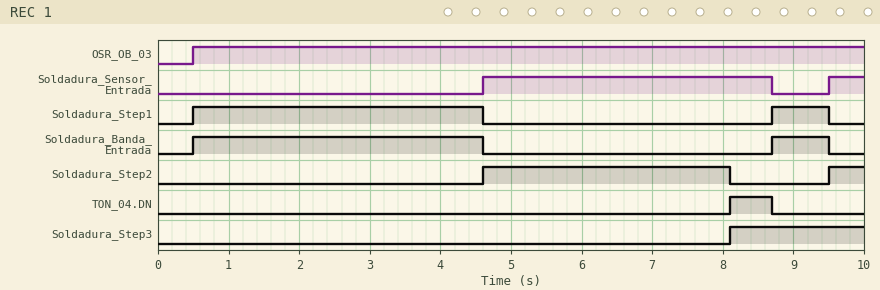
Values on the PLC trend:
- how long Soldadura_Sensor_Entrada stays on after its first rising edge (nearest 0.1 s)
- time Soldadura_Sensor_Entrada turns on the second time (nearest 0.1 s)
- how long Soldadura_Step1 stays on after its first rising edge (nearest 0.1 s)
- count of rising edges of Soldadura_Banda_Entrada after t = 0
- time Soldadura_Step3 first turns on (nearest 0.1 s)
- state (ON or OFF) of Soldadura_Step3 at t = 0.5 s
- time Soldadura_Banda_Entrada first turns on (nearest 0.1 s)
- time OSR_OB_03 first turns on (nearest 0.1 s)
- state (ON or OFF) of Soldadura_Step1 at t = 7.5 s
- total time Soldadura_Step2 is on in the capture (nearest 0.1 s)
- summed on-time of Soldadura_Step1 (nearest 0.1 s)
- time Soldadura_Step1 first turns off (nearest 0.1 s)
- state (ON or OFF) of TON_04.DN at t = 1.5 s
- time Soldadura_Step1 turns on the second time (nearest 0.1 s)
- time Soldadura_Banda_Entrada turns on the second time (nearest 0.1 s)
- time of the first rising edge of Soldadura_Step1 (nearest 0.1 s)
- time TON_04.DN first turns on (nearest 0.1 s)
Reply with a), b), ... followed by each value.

a) 4.1 s
b) 9.5 s
c) 4.1 s
d) 2
e) 8.1 s
f) OFF
g) 0.5 s
h) 0.5 s
i) OFF
j) 4.0 s
k) 4.9 s
l) 4.6 s
m) OFF
n) 8.7 s
o) 8.7 s
p) 0.5 s
q) 8.1 s
